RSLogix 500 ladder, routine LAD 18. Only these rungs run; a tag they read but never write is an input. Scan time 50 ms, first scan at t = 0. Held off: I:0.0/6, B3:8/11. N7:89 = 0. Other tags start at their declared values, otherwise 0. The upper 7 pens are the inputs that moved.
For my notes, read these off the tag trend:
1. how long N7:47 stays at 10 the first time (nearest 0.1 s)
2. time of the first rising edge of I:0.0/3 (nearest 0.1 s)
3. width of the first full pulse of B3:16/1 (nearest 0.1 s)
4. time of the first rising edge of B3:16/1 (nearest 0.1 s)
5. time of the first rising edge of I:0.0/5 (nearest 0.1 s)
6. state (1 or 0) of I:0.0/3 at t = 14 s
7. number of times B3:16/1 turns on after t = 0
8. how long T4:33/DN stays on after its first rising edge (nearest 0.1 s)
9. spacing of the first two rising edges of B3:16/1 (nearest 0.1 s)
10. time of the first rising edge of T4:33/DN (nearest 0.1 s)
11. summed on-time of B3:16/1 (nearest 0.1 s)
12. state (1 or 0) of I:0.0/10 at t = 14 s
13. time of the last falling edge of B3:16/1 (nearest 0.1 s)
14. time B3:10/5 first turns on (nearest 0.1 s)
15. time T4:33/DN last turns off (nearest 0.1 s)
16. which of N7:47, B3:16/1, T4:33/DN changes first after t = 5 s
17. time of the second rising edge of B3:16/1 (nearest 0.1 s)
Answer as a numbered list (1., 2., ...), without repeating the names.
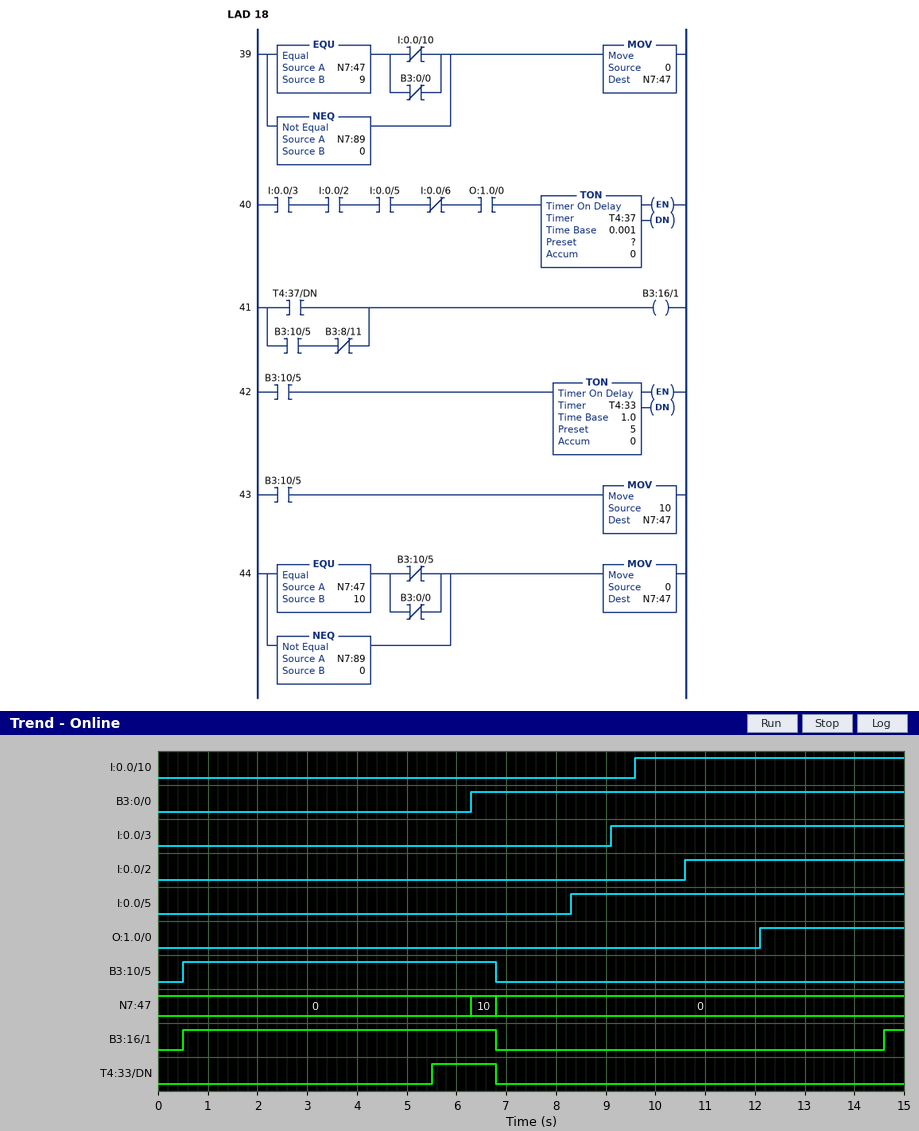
1. 0.5 s
2. 9.1 s
3. 6.3 s
4. 0.5 s
5. 8.3 s
6. 1
7. 2
8. 1.3 s
9. 14.1 s
10. 5.5 s
11. 6.7 s
12. 1
13. 6.8 s
14. 0.5 s
15. 6.8 s
16. T4:33/DN
17. 14.6 s
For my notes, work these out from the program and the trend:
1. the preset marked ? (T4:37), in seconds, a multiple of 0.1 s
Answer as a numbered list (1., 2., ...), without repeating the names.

1. 2.5 s
